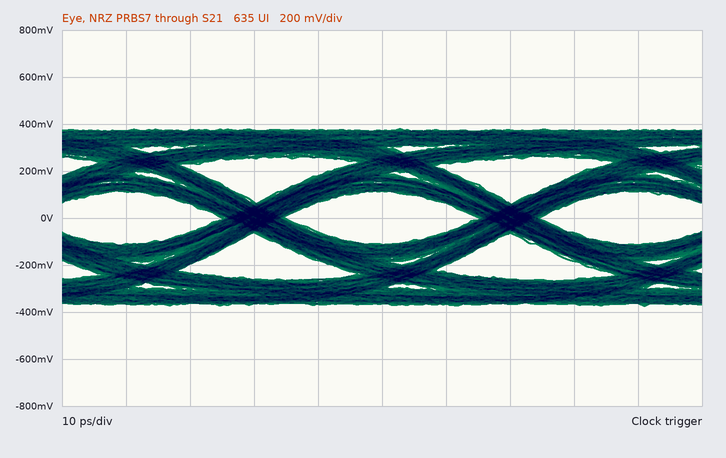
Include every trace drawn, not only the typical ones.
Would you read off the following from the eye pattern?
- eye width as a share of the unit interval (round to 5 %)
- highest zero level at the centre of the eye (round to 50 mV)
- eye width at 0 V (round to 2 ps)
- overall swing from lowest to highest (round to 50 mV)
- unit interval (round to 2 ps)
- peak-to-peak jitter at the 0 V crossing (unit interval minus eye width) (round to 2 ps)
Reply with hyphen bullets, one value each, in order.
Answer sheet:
- 75 %
- -100 mV
- 30 ps
- 750 mV
- 40 ps
- 10 ps
